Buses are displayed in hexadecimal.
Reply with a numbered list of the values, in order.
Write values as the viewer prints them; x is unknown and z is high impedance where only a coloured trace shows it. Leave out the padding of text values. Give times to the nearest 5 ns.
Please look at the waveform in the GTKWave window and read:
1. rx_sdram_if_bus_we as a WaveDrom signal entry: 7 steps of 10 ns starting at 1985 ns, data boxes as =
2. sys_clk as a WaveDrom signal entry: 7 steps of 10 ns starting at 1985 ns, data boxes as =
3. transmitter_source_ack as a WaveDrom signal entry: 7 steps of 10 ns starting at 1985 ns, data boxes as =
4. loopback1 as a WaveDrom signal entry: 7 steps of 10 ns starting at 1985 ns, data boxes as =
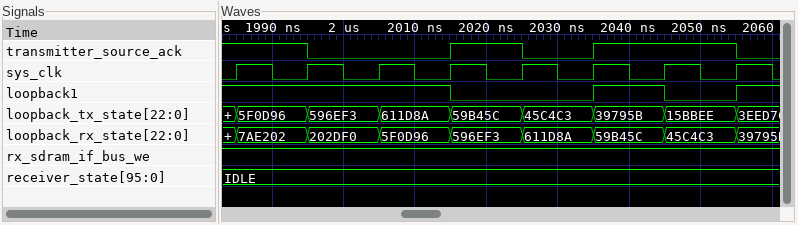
1. {name: 'rx_sdram_if_bus_we', wave: '1......'}
2. {name: 'sys_clk', wave: 'p......'}
3. {name: 'transmitter_source_ack', wave: '10.101.'}
4. {name: 'loopback1', wave: '1..0.10'}
